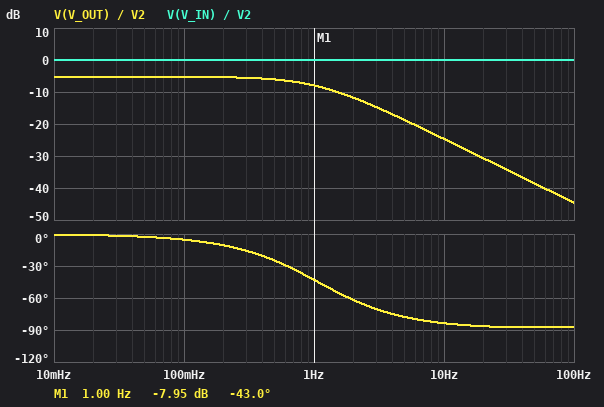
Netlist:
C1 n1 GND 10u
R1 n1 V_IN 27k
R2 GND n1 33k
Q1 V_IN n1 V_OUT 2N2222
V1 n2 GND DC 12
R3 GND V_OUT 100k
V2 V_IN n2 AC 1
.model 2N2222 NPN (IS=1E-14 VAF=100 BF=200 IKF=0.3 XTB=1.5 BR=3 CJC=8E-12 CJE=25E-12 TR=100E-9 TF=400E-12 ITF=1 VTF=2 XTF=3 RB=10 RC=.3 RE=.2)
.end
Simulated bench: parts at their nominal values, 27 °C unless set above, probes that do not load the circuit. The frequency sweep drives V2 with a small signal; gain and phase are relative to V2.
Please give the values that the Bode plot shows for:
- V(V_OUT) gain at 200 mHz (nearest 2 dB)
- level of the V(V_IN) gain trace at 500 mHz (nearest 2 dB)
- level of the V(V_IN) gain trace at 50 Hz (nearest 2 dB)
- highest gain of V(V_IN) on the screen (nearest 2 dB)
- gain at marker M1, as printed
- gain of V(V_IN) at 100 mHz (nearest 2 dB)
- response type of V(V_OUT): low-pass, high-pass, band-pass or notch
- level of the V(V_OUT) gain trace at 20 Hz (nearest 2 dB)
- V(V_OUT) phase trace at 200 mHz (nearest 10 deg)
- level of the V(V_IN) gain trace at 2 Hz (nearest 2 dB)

-6 dB
0 dB
0 dB
0 dB
-7.95 dB
0 dB
low-pass
-30 dB
-10 deg
0 dB
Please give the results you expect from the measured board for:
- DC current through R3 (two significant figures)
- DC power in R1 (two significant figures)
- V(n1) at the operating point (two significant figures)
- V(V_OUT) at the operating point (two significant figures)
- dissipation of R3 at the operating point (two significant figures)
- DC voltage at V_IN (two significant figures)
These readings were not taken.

60 µA
1.1 mW
6.6 V
6.0 V
360 µW
12 V
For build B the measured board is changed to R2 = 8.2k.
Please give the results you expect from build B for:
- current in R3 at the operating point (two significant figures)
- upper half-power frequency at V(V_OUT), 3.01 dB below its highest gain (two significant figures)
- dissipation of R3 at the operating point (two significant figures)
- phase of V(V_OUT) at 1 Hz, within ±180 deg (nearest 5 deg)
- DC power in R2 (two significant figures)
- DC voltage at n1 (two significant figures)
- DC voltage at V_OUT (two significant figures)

22 µA
2.5 Hz
50 µW
-20 deg
950 µW
2.8 V
2.2 V
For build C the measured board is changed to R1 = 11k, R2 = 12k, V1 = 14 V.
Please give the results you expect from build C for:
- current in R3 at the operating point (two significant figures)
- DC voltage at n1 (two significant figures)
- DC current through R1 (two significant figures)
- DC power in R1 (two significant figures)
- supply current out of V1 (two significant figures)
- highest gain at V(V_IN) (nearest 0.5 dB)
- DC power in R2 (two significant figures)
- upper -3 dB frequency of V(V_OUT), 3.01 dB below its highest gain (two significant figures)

67 µA
7.3 V
610 µA
4.1 mW
680 µA
0 dB
4.4 mW
2.8 Hz
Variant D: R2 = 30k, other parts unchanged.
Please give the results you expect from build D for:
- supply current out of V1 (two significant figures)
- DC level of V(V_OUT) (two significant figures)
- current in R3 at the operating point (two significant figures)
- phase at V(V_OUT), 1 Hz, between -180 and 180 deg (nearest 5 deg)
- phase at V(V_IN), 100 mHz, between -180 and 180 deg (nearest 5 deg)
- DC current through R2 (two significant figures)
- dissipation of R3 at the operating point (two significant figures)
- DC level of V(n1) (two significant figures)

270 µA
5.7 V
57 µA
-40 deg
0 deg
210 µA
330 µW
6.3 V
